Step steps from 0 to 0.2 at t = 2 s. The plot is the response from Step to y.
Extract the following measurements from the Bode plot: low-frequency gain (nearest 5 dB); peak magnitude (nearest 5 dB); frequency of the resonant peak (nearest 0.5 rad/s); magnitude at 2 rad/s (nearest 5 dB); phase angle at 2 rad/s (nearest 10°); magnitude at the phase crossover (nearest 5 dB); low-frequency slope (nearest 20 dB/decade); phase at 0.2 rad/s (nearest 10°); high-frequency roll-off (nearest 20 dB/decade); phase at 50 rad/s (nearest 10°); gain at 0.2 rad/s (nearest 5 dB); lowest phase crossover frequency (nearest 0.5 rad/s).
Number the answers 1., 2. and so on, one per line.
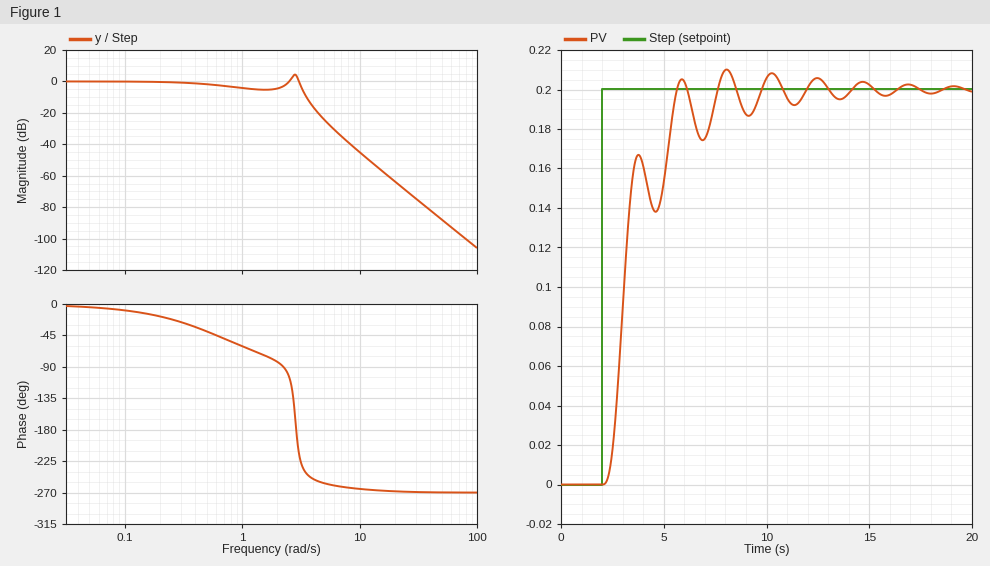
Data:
1. 0 dB
2. 5 dB
3. 3.0 rad/s
4. -5 dB
5. -80°
6. 5 dB
7. 0 dB/decade
8. -20°
9. -60 dB/decade
10. -270°
11. 0 dB
12. 3.0 rad/s
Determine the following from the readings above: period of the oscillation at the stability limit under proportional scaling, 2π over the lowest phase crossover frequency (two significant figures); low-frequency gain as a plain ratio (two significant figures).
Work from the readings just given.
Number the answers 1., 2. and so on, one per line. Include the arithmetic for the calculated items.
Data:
1. 2π / 3 = 2.1 s
2. 10^(0 / 20) = 1.0
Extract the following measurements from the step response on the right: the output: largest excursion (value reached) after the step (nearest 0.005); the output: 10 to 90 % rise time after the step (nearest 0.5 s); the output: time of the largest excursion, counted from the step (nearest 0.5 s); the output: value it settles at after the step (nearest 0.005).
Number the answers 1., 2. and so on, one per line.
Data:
1. 0.210
2. 3.0 s
3. 6.0 s
4. 0.200
